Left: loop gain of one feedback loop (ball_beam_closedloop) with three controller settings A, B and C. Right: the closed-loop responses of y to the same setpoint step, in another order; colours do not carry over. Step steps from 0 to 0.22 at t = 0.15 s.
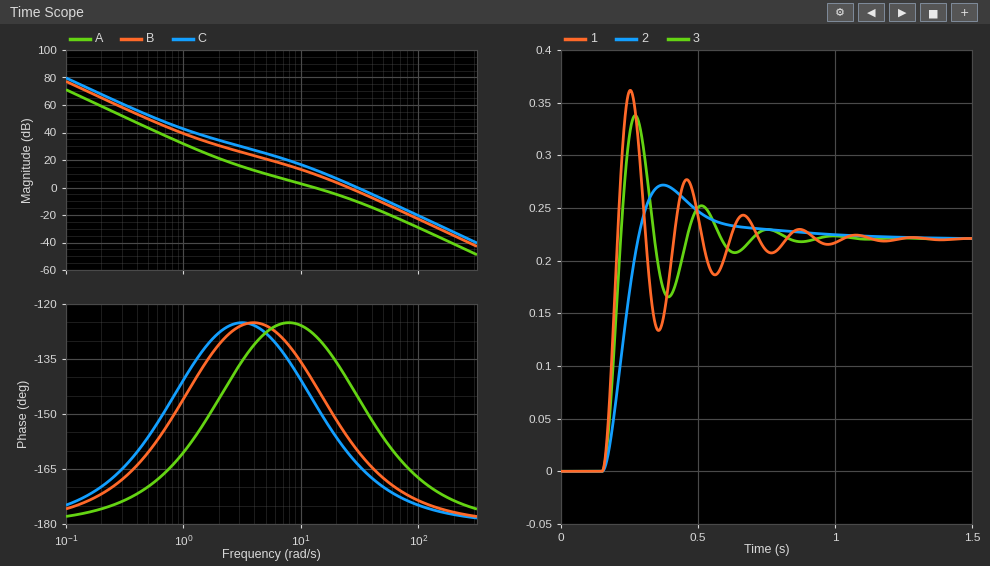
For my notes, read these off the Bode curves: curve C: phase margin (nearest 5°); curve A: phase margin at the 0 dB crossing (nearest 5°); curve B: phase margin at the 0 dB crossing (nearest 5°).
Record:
15°
50°
25°
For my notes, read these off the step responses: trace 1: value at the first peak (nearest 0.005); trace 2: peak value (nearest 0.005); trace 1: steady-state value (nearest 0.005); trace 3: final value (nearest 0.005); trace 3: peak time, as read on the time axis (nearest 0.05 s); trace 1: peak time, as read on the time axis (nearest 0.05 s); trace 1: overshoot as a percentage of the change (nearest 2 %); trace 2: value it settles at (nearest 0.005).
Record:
0.360
0.270
0.220
0.220
0.25 s
0.25 s
64 %
0.220
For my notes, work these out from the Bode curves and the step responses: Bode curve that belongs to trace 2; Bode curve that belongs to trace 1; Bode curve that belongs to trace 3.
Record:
A
C
B
